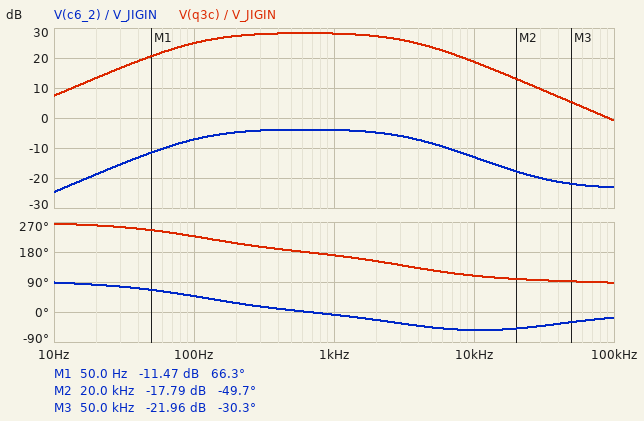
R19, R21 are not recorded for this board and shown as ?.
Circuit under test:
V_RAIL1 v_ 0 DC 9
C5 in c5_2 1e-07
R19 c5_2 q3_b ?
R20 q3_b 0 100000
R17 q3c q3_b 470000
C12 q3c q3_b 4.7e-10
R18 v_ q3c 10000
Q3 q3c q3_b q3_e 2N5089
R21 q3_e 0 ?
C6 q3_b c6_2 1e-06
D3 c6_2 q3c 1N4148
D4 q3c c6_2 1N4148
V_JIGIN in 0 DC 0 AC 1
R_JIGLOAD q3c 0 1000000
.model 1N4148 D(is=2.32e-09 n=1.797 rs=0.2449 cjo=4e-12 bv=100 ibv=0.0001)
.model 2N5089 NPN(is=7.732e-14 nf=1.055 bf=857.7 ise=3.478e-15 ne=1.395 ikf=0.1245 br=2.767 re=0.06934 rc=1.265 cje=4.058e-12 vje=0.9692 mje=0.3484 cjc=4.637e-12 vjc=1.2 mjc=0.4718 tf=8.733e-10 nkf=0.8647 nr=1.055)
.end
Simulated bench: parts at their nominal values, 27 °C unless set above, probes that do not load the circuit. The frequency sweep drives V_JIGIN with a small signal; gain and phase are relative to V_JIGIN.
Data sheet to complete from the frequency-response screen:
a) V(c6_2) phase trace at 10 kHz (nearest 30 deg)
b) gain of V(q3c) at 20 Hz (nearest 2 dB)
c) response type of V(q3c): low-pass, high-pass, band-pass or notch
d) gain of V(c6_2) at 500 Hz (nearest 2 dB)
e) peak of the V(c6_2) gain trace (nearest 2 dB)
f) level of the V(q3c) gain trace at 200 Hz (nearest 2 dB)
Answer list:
-60 deg
14 dB
band-pass
-4 dB
-4 dB
28 dB
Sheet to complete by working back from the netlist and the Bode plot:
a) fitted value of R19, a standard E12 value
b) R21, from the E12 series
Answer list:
3.3 kΩ
180 Ω
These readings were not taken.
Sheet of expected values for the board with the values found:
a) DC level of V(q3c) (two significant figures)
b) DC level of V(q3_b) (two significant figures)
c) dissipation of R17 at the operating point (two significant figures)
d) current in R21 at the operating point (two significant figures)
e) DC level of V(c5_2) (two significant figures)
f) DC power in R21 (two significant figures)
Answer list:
4.3 V
700 mV
27 µW
460 µA
700 mV
38 µW
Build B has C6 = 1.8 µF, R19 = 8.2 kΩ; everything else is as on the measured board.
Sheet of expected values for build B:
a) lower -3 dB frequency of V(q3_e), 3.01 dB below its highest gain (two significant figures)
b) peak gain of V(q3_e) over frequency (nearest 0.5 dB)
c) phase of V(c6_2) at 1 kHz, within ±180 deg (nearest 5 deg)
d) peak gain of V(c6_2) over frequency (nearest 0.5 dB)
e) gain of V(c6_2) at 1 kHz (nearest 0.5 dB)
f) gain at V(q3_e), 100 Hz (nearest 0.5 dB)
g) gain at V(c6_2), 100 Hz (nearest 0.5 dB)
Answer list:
79 Hz
-9.0 dB
-20 deg
-6.5 dB
-7.0 dB
-11.0 dB
-8.5 dB
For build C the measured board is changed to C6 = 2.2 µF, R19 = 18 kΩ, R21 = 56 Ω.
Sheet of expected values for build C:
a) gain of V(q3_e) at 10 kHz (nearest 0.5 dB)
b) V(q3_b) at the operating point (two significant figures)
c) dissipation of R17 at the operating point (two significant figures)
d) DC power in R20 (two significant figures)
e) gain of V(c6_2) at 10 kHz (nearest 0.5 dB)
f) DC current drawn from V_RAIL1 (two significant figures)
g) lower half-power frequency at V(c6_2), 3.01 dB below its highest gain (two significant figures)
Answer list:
-39.5 dB
640 mV
24 µW
4.1 µW
-33.5 dB
500 µA
61 Hz
